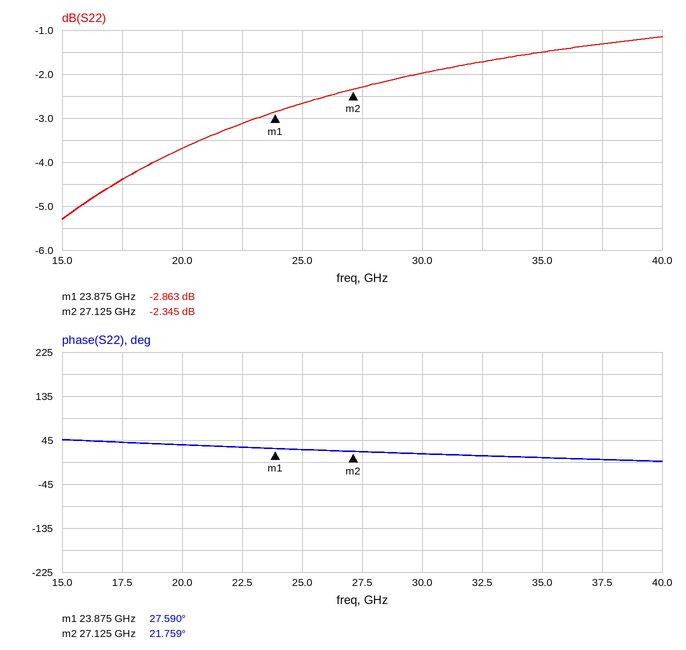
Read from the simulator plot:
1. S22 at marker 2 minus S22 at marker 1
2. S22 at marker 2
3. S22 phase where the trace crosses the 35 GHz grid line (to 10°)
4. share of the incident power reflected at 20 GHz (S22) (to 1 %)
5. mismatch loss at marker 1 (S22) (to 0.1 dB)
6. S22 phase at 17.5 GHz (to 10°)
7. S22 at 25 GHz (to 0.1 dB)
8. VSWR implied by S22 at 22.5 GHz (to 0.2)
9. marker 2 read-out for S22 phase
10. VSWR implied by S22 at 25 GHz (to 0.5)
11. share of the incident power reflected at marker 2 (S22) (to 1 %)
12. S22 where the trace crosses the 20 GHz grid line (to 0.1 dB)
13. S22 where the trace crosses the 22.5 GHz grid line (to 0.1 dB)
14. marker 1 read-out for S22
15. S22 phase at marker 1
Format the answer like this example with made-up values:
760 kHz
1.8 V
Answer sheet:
0.518 dB
-2.345 dB
10°
43 %
3.2 dB
40°
-2.7 dB
5.6
21.759°
6.5
58 %
-3.7 dB
-3.1 dB
-2.863 dB
27.590°
